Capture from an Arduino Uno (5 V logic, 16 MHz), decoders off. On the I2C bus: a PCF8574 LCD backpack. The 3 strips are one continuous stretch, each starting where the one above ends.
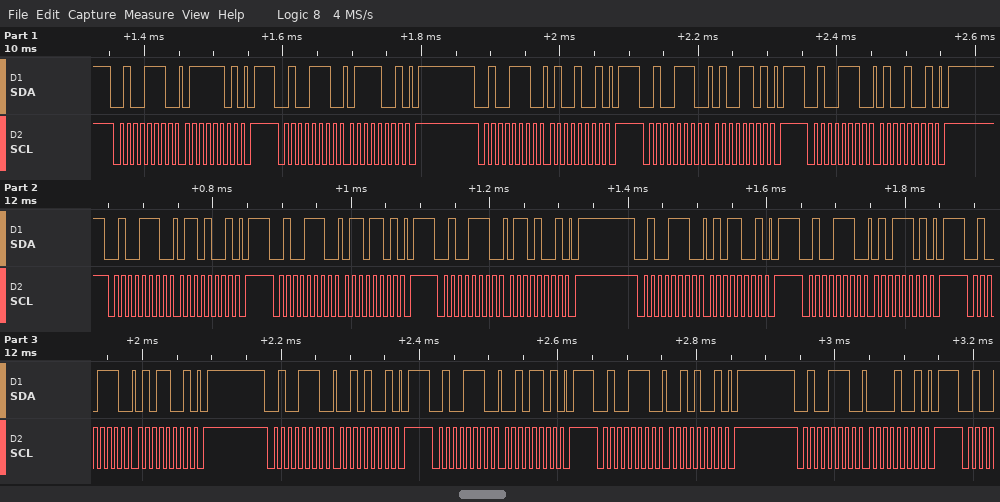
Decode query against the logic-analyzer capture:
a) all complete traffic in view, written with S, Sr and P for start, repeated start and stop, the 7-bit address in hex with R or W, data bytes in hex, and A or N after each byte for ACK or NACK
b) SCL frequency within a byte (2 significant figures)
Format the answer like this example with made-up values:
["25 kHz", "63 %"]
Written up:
["S 27W A 7D A P S 27W A 79 A P S 27W A 49 A P S 27W A 4D A P S 27W A 49 A P S 27W A 69 A P S 27W A 6D A P S 27W A 69 A P S 27W A 59 A P S 27W A 5D A P S 27W A 59 A P S 27W A 29 A P S 27W A 2D A P S 27W A 29 A P S 27W A 09 A P", "100 kHz"]
